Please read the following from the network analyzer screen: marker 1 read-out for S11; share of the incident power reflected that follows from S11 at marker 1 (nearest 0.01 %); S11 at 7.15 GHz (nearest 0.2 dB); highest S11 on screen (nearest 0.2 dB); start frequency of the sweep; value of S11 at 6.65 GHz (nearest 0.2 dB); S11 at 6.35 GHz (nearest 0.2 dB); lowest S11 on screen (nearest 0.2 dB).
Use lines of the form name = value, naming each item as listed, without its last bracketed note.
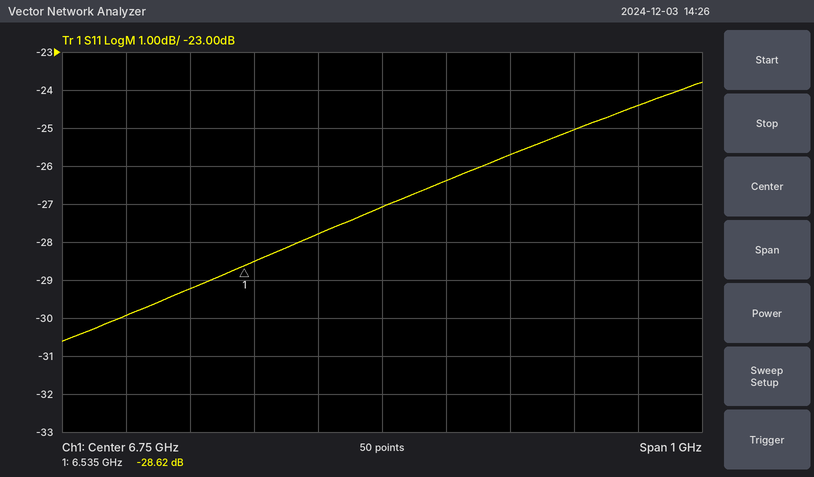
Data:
marker 1 read-out for S11 = -28.62 dB
share of the incident power reflected that follows from S11 at marker 1 = 0.14 %
S11 at 7.15 GHz = -24.4 dB
highest S11 on screen = -23.8 dB
start frequency of the sweep = 6.25 GHz
value of S11 at 6.65 GHz = -27.8 dB
S11 at 6.35 GHz = -30.0 dB
lowest S11 on screen = -30.6 dB
